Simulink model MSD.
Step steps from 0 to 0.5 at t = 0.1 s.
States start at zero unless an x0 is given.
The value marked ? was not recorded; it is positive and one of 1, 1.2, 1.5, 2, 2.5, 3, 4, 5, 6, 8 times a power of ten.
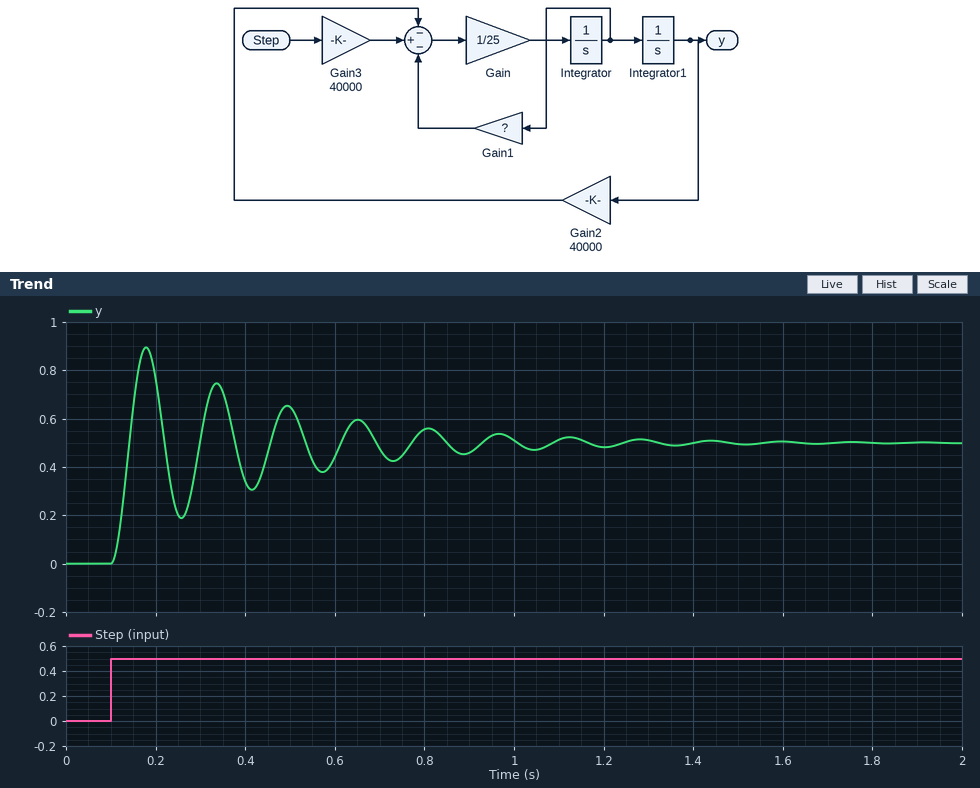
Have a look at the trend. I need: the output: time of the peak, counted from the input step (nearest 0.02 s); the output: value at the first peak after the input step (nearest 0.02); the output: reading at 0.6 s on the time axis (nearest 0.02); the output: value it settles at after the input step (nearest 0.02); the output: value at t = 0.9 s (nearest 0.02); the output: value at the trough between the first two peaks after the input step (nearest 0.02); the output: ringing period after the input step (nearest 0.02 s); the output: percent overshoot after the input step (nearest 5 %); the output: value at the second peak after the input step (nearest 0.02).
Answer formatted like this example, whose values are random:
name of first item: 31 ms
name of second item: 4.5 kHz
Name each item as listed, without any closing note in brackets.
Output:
the output: time of the peak, counted from the input step: 0.08 s
the output: value at the first peak after the input step: 0.90
the output: reading at 0.6 s on the time axis: 0.44
the output: value it settles at after the input step: 0.50
the output: value at t = 0.9 s: 0.46
the output: value at the trough between the first two peaks after the input step: 0.18
the output: ringing period after the input step: 0.16 s
the output: percent overshoot after the input step: 80 %
the output: value at the second peak after the input step: 0.74
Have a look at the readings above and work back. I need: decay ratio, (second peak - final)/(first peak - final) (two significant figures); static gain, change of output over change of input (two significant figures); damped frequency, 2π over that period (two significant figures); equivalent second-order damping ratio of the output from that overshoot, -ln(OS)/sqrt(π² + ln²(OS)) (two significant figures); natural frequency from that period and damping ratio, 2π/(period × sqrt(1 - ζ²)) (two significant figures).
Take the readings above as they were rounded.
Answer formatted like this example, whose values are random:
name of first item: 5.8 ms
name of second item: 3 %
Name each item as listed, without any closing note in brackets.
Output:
decay ratio, (second peak - final)/(first peak - final): 0.60
static gain, change of output over change of input: 1.0
damped frequency, 2π over that period: 39 rad/s
equivalent second-order damping ratio of the output from that overshoot, -ln(OS)/sqrt(π² + ln²(OS)): 0.071
natural frequency from that period and damping ratio, 2π/(period × sqrt(1 - ζ²)): 39 rad/s
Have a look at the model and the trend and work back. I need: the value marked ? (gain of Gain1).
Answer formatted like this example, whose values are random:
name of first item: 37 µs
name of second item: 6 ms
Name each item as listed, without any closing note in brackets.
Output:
the value marked ?: 150
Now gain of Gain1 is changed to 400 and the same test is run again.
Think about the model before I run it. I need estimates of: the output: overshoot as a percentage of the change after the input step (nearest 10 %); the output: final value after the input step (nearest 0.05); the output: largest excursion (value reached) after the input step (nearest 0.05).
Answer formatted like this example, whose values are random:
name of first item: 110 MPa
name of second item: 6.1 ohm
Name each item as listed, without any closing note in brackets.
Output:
the output: overshoot as a percentage of the change after the input step: 50 %
the output: final value after the input step: 0.50
the output: largest excursion (value reached) after the input step: 0.75
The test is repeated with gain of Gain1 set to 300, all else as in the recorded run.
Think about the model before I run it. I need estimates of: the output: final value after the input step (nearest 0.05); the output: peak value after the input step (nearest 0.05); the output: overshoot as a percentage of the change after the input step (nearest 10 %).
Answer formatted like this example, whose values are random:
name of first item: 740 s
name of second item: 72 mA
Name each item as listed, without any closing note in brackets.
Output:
the output: final value after the input step: 0.50
the output: peak value after the input step: 0.80
the output: overshoot as a percentage of the change after the input step: 60 %
